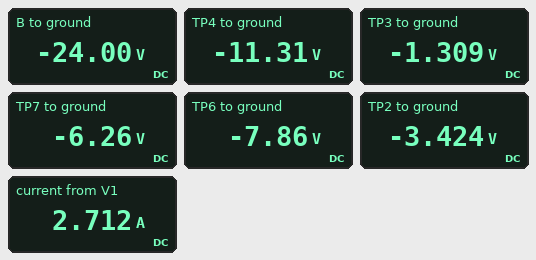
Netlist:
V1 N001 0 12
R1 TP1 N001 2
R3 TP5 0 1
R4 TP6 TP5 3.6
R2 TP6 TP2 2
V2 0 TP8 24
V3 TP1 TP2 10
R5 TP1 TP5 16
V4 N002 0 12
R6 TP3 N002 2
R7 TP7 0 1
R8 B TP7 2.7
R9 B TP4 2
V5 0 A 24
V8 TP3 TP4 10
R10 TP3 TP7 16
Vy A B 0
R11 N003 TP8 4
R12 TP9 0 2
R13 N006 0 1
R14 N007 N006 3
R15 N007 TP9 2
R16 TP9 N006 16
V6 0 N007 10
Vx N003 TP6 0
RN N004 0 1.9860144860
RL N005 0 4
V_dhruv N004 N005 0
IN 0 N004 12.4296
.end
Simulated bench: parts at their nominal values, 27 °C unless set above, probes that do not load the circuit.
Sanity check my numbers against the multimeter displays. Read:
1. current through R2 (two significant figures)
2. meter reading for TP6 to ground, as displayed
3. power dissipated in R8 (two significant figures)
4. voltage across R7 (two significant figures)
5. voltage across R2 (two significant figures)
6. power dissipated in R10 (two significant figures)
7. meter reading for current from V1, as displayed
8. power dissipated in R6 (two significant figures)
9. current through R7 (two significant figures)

2.2 A
-7.86 V
120 W
6.3 V
4.4 V
1.5 W
2.712 A
89 W
6.3 A
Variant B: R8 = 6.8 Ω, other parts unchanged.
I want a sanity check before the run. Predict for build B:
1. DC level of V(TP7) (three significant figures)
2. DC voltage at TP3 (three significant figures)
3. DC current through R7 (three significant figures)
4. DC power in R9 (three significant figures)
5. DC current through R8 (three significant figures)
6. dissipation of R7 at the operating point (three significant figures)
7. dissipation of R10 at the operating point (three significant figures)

-2.98 V
-1.12 V
2.98 A
83.0 W
3.09 A
8.85 W
216 mW
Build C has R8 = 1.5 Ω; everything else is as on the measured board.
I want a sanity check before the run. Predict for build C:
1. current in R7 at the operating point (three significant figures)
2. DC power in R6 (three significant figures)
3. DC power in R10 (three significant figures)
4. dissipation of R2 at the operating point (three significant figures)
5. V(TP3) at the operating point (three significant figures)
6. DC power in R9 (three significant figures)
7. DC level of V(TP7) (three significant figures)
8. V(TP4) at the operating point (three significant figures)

9.31 A
91.0 W
3.82 W
9.84 W
-1.49 V
78.3 W
-9.31 V
-11.5 V
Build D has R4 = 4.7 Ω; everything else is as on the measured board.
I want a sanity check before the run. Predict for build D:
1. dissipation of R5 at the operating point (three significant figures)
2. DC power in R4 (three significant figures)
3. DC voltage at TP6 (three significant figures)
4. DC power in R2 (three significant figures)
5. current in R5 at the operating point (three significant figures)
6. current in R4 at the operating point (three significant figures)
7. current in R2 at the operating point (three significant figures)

3.46 W
11.3 W
-8.37 V
11.1 W
465 mA
1.55 A
2.36 A
